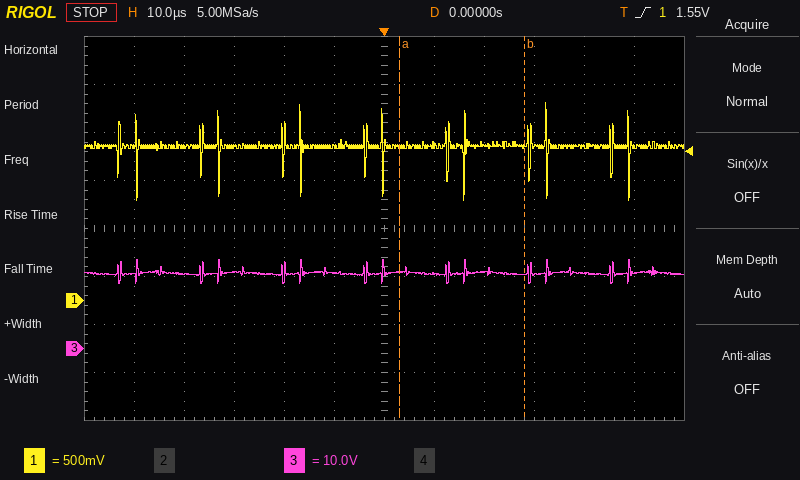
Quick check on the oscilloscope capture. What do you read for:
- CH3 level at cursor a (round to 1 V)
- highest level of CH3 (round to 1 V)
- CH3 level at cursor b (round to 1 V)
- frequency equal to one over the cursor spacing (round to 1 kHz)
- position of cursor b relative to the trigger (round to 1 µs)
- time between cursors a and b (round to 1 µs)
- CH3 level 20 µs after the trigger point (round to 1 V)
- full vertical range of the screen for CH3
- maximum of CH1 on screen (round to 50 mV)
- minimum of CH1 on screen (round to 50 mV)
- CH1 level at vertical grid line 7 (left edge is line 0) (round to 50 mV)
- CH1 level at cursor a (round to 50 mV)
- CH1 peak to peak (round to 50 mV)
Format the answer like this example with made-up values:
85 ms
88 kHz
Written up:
16 V
19 V
16 V
40 kHz
+28 µs
25 µs
16 V
80 V
2.05 V
1.05 V
1.60 V
1.60 V
1.00 V
